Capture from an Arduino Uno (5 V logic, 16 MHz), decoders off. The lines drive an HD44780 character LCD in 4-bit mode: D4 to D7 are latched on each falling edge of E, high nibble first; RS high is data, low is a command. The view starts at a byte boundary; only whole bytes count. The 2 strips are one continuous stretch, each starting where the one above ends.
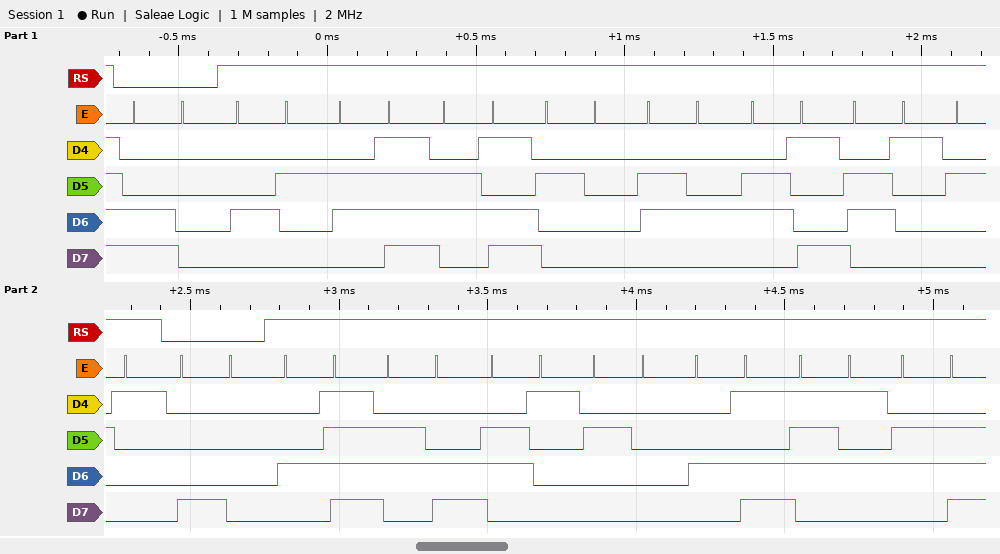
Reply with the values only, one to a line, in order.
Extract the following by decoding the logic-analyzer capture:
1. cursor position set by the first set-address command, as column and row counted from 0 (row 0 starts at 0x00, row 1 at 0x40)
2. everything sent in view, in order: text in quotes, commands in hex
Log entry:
column 0, row 1
0xC0 "Bom dia!" 0x80 "Ola Mun"
